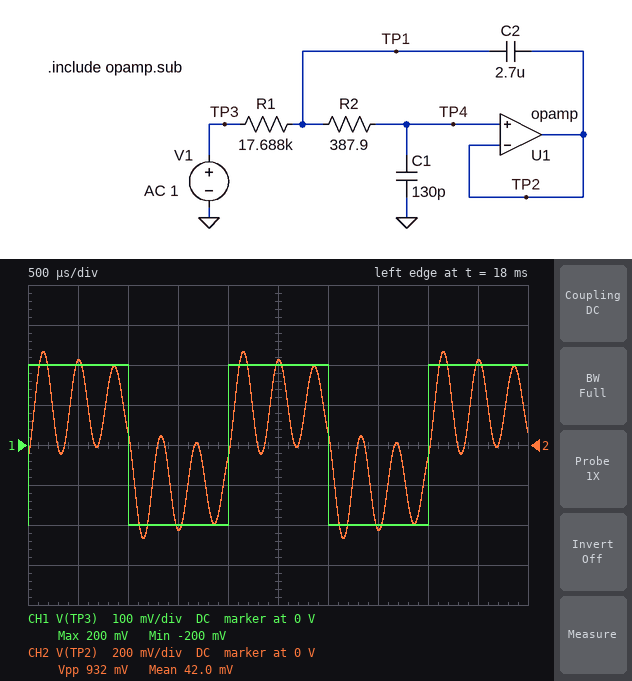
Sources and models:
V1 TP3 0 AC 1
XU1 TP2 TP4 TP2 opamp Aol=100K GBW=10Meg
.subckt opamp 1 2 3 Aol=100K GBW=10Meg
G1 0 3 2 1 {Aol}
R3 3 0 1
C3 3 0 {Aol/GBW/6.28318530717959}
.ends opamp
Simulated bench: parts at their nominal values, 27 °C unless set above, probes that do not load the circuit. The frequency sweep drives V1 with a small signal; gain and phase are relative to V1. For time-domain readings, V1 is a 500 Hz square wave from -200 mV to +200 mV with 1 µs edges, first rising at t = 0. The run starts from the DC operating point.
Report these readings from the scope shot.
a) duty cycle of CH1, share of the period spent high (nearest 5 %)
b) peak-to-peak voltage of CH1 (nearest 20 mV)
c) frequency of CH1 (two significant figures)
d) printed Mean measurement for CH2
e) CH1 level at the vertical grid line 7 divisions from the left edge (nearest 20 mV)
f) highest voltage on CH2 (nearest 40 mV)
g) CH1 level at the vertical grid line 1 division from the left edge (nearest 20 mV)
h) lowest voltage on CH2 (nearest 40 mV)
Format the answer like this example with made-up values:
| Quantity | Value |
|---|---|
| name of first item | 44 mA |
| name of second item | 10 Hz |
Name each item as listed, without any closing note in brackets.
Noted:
| Quantity | Value |
|---|---|
| duty cycle of CH1, share of the period spent high | 50 % |
| peak-to-peak voltage of CH1 | 400 mV |
| frequency of CH1 | 500 Hz |
| printed Mean measurement for CH2 | 42.0 mV |
| CH1 level at the vertical grid line 7 divisions from the left edge | -200 mV |
| highest voltage on CH2 | 480 mV |
| CH1 level at the vertical grid line 1 division from the left edge | 200 mV |
| lowest voltage on CH2 | -480 mV |
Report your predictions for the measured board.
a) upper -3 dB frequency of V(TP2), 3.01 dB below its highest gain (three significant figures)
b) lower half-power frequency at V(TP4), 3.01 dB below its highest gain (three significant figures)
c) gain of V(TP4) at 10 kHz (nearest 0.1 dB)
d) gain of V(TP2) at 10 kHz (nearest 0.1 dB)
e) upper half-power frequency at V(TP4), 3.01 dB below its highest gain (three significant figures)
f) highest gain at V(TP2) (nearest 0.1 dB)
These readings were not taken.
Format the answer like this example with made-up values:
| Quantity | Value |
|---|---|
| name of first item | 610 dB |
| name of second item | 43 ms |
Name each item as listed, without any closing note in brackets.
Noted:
| Quantity | Value |
|---|---|
| upper -3 dB frequency of V(TP2), 3.01 dB below its highest gain | 2.90 kHz |
| lower half-power frequency at V(TP4), 3.01 dB below its highest gain | 2.75 kHz |
| gain of V(TP4) at 10 kHz | -21.2 dB |
| gain of V(TP2) at 10 kHz | -21.2 dB |
| upper half-power frequency at V(TP4), 3.01 dB below its highest gain | 2.90 kHz |
| highest gain at V(TP2) | 26.0 dB |
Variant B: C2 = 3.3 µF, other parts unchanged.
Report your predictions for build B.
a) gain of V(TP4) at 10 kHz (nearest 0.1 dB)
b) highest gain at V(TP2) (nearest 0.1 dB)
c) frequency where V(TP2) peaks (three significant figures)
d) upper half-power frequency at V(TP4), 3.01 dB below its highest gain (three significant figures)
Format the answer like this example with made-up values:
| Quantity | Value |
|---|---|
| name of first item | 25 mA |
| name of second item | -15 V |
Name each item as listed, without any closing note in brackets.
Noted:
| Quantity | Value |
|---|---|
| gain of V(TP4) at 10 kHz | -23.1 dB |
| highest gain at V(TP2) | 26.5 dB |
| frequency where V(TP2) peaks | 2.56 kHz |
| upper half-power frequency at V(TP4), 3.01 dB below its highest gain | 2.62 kHz |
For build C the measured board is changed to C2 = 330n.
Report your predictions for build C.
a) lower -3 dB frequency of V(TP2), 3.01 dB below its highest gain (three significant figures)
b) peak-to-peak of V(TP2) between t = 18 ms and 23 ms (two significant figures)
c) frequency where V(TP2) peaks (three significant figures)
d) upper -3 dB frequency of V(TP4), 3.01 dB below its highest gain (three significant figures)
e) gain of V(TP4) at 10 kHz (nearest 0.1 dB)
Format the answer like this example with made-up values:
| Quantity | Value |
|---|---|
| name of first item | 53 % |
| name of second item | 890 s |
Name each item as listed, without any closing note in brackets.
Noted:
| Quantity | Value |
|---|---|
| lower -3 dB frequency of V(TP2), 3.01 dB below its highest gain | 7.54 kHz |
| peak-to-peak of V(TP2) between t = 18 ms and 23 ms | 1.0 V |
| frequency where V(TP2) peaks | 8.06 kHz |
| upper -3 dB frequency of V(TP4), 3.01 dB below its highest gain | 8.54 kHz |
| gain of V(TP4) at 10 kHz | 5.2 dB |
